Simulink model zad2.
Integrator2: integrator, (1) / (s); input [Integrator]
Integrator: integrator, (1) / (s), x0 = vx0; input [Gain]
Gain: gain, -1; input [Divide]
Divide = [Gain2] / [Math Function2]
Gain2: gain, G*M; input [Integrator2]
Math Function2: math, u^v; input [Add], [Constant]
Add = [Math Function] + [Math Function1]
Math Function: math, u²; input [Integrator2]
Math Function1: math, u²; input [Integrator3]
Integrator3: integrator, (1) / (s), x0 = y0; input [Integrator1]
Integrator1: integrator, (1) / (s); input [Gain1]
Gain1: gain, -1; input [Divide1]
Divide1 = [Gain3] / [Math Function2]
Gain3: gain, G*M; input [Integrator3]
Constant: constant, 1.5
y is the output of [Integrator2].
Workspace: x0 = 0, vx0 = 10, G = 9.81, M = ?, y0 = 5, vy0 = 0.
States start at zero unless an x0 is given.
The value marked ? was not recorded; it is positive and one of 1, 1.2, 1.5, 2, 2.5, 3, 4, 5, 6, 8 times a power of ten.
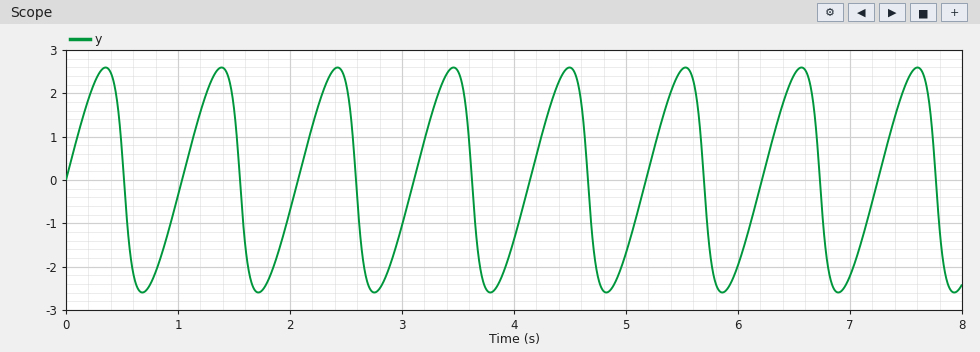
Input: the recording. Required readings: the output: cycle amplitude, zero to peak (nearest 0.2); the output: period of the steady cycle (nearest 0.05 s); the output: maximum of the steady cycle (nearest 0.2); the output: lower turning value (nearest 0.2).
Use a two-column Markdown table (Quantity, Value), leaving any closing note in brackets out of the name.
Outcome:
| Quantity | Value |
|---|---|
| the output: cycle amplitude, zero to peak | 2.6 |
| the output: period of the steady cycle | 1.05 s |
| the output: maximum of the steady cycle | 2.6 |
| the output: lower turning value | -2.6 |
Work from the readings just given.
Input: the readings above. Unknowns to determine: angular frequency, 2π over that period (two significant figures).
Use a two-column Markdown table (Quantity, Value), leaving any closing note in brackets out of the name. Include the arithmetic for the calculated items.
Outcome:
| Quantity | Value |
|---|---|
| angular frequency, 2π over that period | 2π / 1.05 = 6.0 rad/s |
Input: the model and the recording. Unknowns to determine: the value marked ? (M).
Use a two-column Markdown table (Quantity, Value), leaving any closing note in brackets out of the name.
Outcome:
| Quantity | Value |
|---|---|
| the value marked ? | 120 |
